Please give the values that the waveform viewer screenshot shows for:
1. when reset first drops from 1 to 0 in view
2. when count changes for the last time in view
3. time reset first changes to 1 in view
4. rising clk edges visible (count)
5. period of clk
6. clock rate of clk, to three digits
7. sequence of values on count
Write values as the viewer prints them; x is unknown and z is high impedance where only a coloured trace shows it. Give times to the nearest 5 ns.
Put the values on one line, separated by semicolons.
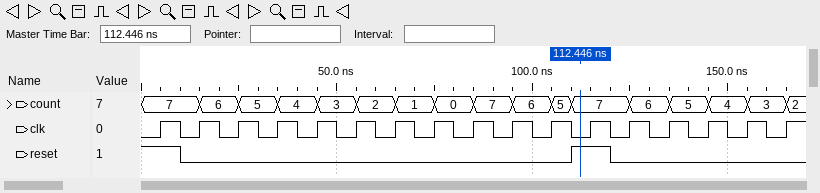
10 ns; 165 ns; 110 ns; 17; 10 ns; 100 MHz; 7, 6, 5, 4, 3, 2, 1, 0, 7, 6, 5, 7, 6, 5, 4, 3, 2
